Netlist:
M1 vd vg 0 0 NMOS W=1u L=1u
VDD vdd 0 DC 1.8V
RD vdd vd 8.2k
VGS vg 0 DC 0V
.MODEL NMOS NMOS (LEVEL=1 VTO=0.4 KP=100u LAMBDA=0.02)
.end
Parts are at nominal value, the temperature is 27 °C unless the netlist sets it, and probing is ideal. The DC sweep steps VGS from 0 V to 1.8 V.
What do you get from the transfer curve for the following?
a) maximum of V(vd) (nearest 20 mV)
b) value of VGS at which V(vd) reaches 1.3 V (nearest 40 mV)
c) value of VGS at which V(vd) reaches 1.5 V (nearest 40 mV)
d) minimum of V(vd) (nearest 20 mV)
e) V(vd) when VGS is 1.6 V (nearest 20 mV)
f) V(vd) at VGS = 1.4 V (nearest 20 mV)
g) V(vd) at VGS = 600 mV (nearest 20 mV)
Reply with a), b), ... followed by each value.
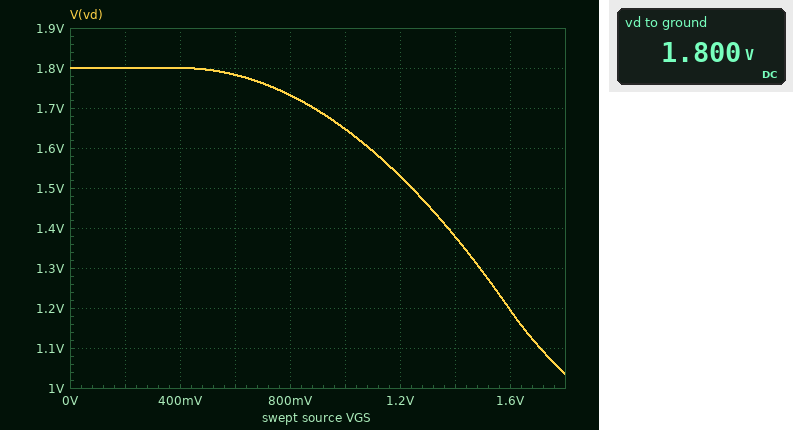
a) 1.80 V
b) 1.48 V
c) 1.24 V
d) 1.04 V
e) 1.20 V
f) 1.38 V
g) 1.78 V
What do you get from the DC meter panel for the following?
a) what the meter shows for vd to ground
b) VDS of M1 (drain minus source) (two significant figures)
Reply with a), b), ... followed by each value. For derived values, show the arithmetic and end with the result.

a) 1.800 V
b) 1.8 V = 1.8 V
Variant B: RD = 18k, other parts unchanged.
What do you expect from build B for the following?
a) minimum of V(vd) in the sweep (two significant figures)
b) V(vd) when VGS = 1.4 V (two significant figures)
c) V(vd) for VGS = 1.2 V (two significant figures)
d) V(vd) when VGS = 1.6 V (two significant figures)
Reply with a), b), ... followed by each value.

a) 600 mV
b) 890 mV
c) 1.2 V
d) 710 mV
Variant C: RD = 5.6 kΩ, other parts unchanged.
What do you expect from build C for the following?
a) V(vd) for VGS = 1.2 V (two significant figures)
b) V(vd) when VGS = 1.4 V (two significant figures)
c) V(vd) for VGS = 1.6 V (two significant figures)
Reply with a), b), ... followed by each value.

a) 1.6 V
b) 1.5 V
c) 1.4 V
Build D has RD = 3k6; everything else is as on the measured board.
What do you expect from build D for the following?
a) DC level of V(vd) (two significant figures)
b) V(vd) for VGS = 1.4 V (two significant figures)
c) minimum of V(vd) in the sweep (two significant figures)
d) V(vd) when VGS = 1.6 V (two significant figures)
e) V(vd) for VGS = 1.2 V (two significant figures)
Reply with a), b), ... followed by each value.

a) 1.8 V
b) 1.6 V
c) 1.4 V
d) 1.5 V
e) 1.7 V
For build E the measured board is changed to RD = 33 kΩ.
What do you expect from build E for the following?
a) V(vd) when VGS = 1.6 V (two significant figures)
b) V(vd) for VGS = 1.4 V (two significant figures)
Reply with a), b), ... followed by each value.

a) 420 mV
b) 520 mV
